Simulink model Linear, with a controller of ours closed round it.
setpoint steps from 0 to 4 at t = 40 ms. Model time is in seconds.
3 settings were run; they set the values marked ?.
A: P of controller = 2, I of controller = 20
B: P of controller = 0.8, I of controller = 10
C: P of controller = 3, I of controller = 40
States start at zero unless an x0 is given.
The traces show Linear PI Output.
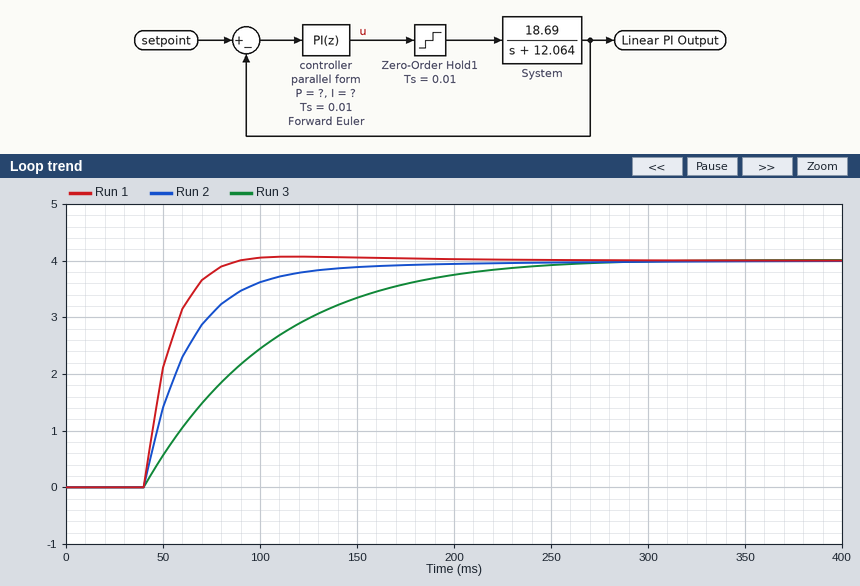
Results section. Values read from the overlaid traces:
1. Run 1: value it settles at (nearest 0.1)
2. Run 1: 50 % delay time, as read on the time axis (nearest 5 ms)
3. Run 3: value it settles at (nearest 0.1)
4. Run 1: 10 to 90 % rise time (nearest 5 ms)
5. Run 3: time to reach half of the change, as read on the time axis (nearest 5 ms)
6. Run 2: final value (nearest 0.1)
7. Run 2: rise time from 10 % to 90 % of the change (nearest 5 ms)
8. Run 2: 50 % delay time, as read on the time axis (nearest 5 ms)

4.0
50 ms
4.0
25 ms
85 ms
4.0
55 ms
55 ms
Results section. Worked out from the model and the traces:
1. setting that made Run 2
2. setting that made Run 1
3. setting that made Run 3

A
C
B
